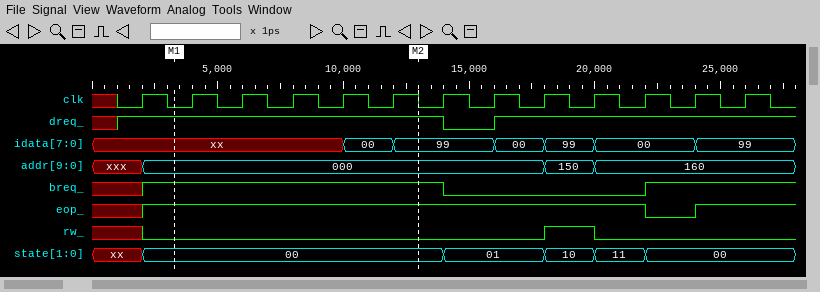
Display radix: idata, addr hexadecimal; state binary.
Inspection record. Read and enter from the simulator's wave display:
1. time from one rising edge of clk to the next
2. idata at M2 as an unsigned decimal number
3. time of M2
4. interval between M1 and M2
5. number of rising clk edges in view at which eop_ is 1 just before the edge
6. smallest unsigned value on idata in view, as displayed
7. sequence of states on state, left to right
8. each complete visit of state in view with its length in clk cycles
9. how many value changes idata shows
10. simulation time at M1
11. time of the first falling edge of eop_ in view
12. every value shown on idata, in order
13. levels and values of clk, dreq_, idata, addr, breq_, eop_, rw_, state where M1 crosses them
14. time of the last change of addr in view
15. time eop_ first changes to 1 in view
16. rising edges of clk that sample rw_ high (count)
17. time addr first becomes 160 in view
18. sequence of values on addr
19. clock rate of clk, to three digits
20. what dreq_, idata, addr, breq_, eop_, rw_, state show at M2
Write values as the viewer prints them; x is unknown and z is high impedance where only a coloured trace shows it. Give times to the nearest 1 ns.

2 ns
153
13 ns
10 ns
11
00
xx, 00, 01, 10, 11, 00
00: 6, 01: 2, 10: 1, 11: 1
6
3 ns
22 ns
xx, 00, 99, 00, 99, 00, 99
clk=0, dreq_=1, idata=xx, addr=000, breq_=1, eop_=1, rw_=0, state=00
20 ns
2 ns
1
20 ns
xxx, 000, 150, 160
500 MHz
dreq_=1, idata=99, addr=000, breq_=1, eop_=1, rw_=0, state=00
